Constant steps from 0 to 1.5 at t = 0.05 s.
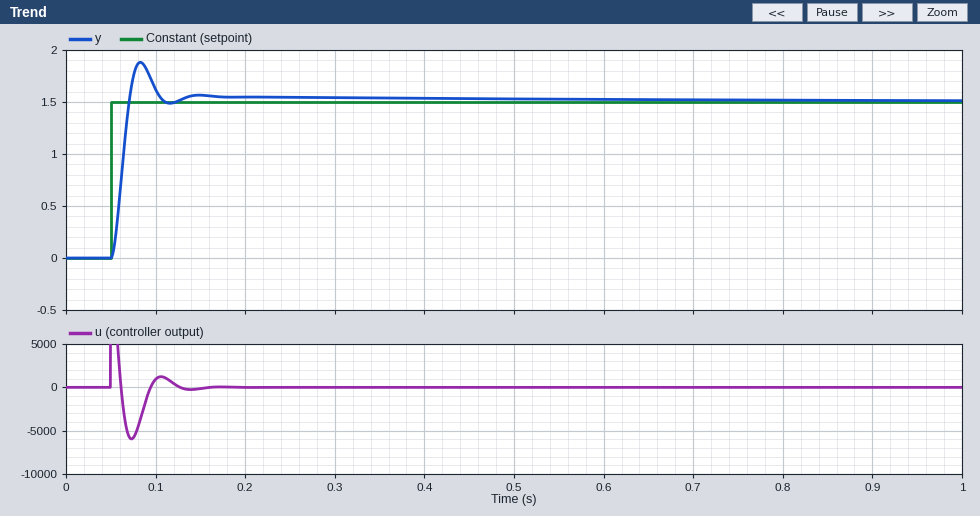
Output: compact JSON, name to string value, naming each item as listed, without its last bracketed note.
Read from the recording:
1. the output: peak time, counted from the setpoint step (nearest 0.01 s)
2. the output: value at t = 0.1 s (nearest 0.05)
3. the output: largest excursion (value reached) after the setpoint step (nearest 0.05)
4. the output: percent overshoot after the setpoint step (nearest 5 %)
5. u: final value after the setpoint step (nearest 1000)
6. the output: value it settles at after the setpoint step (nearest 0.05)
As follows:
{"the output: peak time, counted from the setpoint step": "0.03 s", "the output: value at t = 0.1 s": "1.60", "the output: largest excursion (value reached) after the setpoint step": "1.90", "the output: percent overshoot after the setpoint step": "25 %", "u: final value after the setpoint step": "0", "the output: value it settles at after the setpoint step": "1.50"}
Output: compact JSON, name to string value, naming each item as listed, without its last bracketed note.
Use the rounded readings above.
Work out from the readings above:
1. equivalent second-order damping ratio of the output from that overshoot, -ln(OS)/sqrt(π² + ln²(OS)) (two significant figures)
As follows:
{"equivalent second-order damping ratio of the output from that overshoot, -ln(OS)/sqrt(π² + ln²(OS))": "0.40"}
